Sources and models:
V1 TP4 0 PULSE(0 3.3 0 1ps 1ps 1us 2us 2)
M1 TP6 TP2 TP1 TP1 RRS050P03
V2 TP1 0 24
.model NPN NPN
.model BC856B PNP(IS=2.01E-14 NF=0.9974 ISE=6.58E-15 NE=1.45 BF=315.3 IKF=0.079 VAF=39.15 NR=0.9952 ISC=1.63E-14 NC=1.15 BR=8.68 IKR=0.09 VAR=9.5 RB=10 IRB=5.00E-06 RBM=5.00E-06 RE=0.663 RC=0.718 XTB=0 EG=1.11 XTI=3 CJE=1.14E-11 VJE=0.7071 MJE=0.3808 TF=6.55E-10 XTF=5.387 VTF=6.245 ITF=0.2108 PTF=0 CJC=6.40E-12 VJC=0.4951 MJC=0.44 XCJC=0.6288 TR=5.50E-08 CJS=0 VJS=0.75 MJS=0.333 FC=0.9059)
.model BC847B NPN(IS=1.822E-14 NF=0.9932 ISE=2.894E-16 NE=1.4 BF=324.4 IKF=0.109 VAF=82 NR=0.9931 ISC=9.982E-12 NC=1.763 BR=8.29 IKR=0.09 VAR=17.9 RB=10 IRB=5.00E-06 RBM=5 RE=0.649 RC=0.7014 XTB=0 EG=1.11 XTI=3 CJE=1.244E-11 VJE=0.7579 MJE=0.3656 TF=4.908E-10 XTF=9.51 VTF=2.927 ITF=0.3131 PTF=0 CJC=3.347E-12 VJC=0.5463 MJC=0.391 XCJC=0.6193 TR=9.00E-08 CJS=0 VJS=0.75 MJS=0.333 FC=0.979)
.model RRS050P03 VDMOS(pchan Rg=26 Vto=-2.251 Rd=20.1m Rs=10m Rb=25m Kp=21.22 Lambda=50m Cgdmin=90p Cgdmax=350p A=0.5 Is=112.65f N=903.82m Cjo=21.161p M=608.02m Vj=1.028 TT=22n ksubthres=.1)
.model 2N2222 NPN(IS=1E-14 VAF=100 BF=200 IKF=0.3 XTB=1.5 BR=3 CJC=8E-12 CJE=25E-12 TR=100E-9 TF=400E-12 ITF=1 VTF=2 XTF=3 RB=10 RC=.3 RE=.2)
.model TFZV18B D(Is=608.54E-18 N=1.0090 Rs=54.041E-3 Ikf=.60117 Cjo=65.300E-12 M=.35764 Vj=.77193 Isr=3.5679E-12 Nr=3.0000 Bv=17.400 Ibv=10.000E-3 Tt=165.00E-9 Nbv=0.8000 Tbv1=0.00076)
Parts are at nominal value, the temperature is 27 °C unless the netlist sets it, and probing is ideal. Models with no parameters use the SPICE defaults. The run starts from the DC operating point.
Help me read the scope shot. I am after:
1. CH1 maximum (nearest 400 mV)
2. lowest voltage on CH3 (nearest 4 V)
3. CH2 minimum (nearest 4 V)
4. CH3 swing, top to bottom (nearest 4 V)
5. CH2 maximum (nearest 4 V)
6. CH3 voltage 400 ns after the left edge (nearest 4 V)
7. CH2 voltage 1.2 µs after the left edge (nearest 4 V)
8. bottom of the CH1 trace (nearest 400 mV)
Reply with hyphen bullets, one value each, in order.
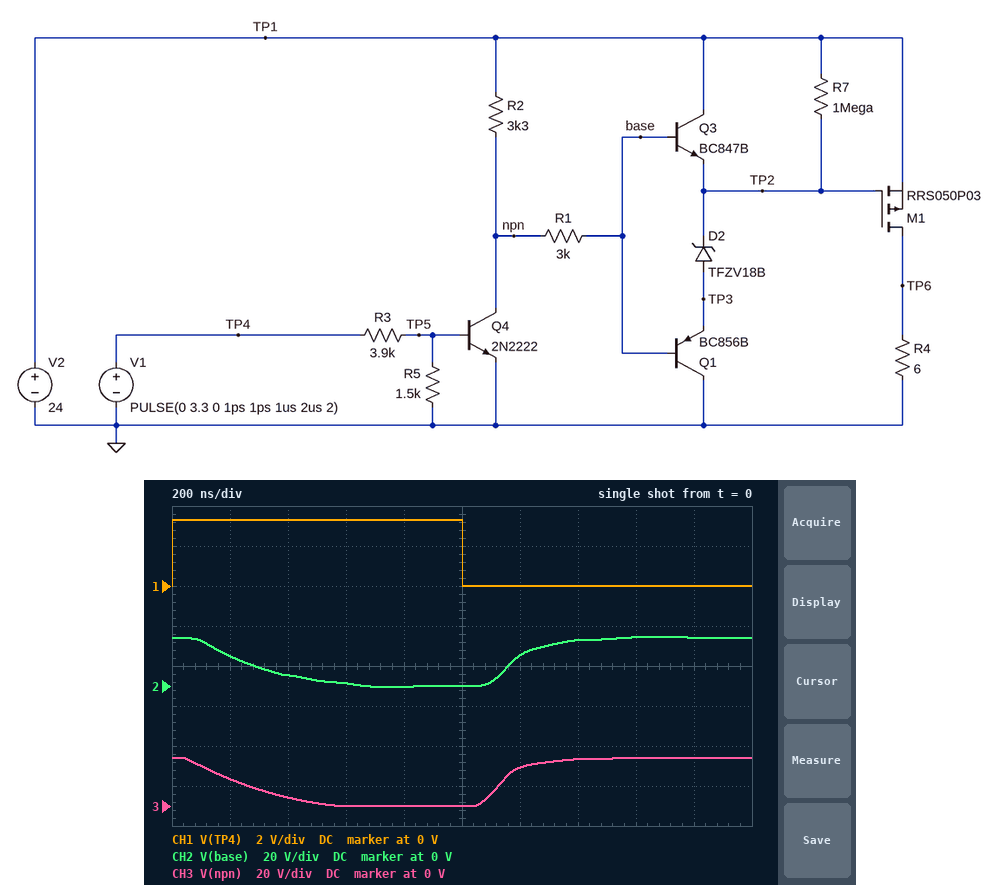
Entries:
- 3.2 V
- 0 V
- 0 V
- 24 V
- 24 V
- 4 V
- 16 V
- 0 V
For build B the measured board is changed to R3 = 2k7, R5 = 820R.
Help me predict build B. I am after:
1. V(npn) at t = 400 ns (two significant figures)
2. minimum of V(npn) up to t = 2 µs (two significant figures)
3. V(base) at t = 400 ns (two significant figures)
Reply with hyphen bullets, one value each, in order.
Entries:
- 9.5 V
- 610 mV
- 10 V
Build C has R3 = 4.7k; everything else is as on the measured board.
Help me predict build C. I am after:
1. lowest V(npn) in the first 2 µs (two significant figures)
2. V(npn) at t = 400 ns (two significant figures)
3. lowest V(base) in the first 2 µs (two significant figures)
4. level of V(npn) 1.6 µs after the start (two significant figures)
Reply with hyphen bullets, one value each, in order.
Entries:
- 3.3 V
- 13 V
- 3.6 V
- 24 V
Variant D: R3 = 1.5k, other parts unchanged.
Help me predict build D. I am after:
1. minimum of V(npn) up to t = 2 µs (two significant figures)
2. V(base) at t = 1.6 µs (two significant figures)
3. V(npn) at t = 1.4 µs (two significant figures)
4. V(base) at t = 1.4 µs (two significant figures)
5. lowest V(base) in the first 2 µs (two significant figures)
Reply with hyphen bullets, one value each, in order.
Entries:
- 32 mV
- 23 V
- 21 V
- 18 V
- -550 mV
